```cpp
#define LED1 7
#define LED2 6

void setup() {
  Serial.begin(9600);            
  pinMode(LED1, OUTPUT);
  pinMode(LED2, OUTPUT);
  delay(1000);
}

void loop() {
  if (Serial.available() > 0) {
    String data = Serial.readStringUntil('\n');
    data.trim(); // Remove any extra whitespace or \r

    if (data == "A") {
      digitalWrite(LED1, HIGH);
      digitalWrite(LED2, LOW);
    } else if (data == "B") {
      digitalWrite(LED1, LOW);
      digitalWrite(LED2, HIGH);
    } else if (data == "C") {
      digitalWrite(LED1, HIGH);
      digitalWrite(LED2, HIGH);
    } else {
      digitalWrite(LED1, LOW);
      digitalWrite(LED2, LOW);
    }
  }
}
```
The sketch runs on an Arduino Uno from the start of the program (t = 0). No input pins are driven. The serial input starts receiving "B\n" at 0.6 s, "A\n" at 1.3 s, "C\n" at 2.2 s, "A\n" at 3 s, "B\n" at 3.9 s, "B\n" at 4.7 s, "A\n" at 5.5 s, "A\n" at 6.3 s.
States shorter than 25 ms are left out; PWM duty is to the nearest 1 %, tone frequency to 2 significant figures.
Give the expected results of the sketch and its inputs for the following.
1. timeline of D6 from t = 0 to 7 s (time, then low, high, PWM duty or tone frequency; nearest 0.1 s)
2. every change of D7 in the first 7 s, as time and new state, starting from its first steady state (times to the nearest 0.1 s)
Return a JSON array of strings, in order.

["0 s low; 1 s high; 1.3 s low; 2.2 s high; 3 s low; 3.9 s high; 5.5 s low", "0 s low; 1.3 s high; 3.9 s low; 5.5 s high"]
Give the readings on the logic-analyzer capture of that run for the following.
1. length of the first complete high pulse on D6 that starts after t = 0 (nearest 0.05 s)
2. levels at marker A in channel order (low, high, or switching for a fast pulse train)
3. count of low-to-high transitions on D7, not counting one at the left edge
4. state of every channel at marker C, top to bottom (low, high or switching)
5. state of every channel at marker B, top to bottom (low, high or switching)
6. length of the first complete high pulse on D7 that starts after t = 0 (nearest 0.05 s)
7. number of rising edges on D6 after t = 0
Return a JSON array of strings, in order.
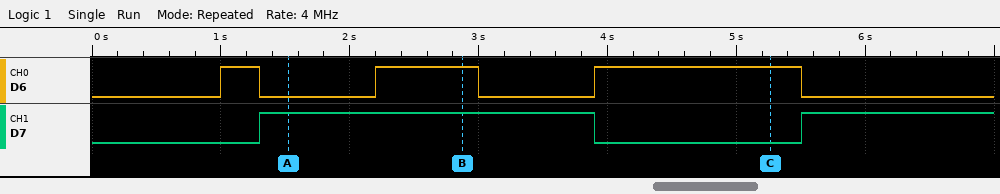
["0.30 s", "D6 low, D7 high", "2", "D6 high, D7 low", "D6 high, D7 high", "2.60 s", "3"]
